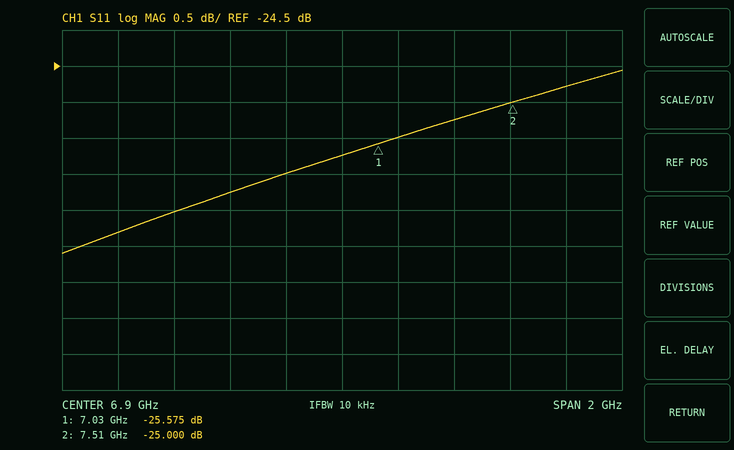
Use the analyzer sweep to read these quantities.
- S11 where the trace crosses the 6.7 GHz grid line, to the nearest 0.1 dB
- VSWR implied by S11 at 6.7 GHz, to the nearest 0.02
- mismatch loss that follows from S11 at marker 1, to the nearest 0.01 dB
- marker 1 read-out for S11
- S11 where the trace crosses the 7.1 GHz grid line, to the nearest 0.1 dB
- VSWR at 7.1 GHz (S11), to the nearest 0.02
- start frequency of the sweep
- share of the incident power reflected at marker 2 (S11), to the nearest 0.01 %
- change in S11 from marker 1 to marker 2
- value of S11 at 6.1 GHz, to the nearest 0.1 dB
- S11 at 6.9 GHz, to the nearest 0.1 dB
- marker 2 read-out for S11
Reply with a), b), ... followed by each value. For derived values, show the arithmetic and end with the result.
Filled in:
a) -26.0 dB
b) |Γ| = 10^(-26/20) = 0.0501; VSWR = (1 + 0.0501)/(1 − 0.0501) ≈ 1.11, so 1.10 to the nearest 0.02
c) −10 log10(1 − 10^(-25.575/10)) ≈ 0.01 dB
d) -25.575 dB
e) -25.5 dB
f) |Γ| = 10^(-25.5/20) = 0.0531; VSWR = (1 + 0.0531)/(1 − 0.0531) ≈ 1.11, so 1.12 to the nearest 0.02
g) 5.9 GHz
h) 10^(-25/10) ≈ 0.32 %
i) -25 − (-25.575) = 0.575 dB
j) -26.8 dB
k) -25.7 dB
l) -25.000 dB
